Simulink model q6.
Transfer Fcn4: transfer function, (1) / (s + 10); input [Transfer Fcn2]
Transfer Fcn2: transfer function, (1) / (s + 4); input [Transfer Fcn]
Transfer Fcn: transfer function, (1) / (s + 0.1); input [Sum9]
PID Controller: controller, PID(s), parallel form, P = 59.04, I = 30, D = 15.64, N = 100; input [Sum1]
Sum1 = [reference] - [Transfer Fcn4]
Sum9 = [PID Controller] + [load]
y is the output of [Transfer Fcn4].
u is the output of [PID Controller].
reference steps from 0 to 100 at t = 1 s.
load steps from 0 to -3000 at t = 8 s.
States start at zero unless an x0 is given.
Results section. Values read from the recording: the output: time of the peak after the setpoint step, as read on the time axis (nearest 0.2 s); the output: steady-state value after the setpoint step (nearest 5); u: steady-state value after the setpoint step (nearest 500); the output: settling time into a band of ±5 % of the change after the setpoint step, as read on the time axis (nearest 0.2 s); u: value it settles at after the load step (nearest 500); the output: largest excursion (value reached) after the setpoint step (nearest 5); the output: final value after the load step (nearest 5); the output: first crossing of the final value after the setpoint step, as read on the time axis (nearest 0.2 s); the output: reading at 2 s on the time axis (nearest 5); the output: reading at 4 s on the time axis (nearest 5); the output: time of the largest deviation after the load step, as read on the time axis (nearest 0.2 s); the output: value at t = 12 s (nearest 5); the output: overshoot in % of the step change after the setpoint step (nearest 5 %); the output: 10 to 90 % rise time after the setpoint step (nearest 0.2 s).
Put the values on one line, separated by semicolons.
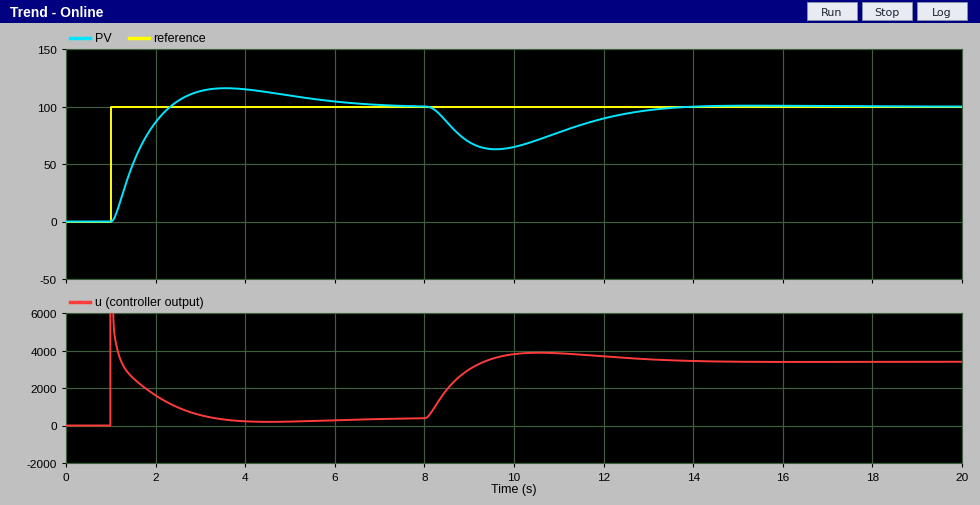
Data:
3.6 s; 100; 500; 5.8 s; 3500; 115; 100; 2.4 s; 85; 115; 9.6 s; 90; 15 %; 1.0 s
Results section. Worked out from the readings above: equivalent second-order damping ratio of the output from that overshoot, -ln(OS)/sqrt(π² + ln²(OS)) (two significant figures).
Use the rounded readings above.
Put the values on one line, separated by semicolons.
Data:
0.52
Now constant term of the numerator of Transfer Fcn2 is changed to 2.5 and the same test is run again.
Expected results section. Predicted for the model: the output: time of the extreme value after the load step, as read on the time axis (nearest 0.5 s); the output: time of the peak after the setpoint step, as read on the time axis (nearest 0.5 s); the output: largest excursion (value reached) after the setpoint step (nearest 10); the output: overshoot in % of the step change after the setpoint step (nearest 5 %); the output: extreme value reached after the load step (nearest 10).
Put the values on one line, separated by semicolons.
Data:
9.0 s; 2.5 s; 110; 10 %; 60
